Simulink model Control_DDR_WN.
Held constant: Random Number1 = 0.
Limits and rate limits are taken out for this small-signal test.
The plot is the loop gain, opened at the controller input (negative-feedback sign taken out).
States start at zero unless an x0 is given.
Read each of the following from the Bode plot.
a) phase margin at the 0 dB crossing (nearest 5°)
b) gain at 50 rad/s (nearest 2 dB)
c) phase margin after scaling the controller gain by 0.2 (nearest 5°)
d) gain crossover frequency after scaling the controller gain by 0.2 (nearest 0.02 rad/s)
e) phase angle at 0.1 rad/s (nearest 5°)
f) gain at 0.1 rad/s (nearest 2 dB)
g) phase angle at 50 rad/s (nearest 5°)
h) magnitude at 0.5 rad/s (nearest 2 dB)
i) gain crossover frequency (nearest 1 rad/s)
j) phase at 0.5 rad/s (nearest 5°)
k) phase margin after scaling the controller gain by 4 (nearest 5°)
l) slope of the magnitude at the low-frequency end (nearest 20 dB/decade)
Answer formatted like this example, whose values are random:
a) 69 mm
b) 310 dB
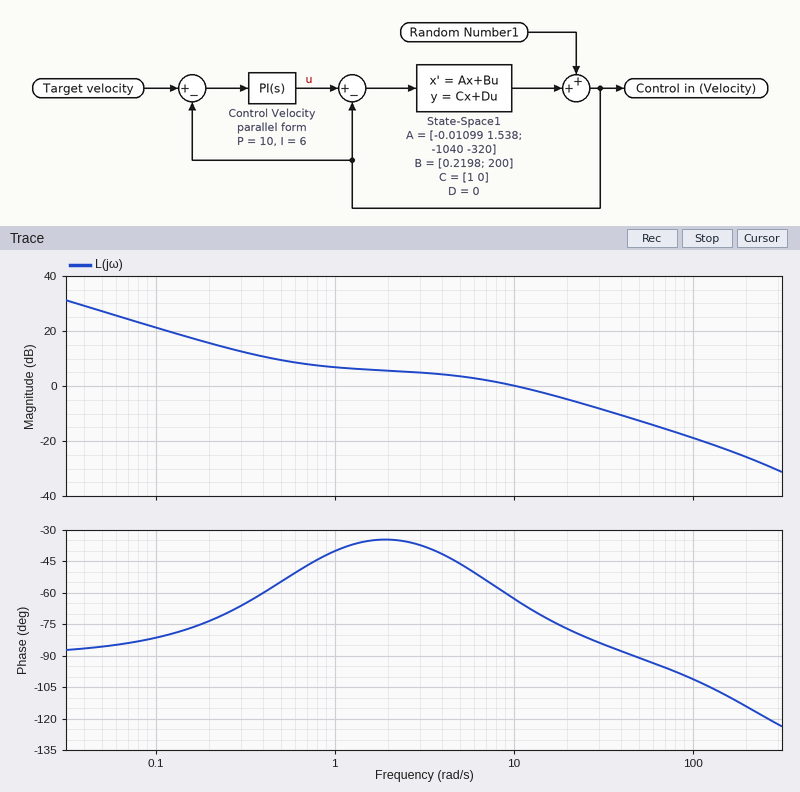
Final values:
a) 115°
b) -12 dB
c) 110°
d) 0.24 rad/s
e) -80°
f) 22 dB
g) -90°
h) 10 dB
i) 10 rad/s
j) -55°
k) 90°
l) -20 dB/decade
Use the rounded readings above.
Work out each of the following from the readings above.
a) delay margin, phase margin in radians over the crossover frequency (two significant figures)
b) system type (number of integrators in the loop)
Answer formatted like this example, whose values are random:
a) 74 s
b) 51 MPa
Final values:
a) 0.20 s
b) 1
